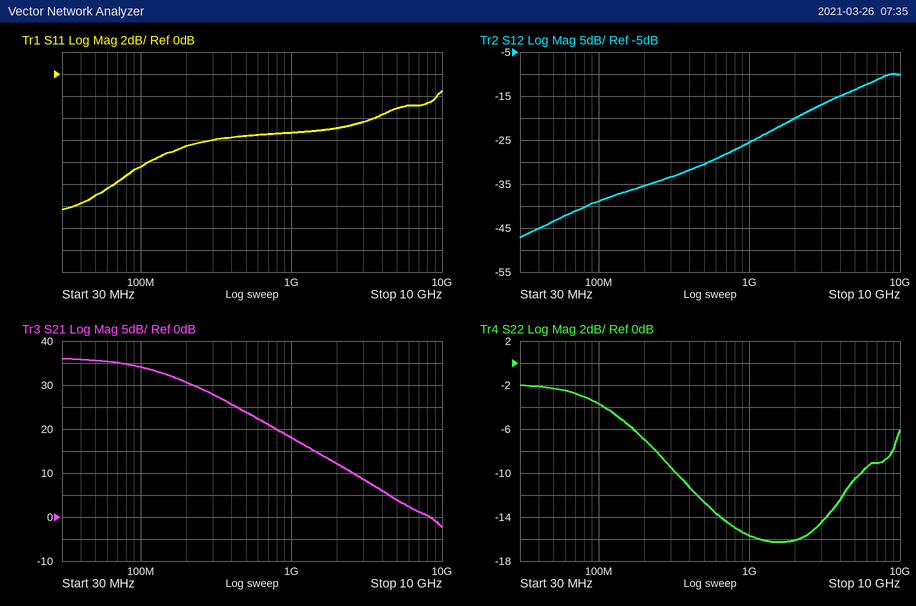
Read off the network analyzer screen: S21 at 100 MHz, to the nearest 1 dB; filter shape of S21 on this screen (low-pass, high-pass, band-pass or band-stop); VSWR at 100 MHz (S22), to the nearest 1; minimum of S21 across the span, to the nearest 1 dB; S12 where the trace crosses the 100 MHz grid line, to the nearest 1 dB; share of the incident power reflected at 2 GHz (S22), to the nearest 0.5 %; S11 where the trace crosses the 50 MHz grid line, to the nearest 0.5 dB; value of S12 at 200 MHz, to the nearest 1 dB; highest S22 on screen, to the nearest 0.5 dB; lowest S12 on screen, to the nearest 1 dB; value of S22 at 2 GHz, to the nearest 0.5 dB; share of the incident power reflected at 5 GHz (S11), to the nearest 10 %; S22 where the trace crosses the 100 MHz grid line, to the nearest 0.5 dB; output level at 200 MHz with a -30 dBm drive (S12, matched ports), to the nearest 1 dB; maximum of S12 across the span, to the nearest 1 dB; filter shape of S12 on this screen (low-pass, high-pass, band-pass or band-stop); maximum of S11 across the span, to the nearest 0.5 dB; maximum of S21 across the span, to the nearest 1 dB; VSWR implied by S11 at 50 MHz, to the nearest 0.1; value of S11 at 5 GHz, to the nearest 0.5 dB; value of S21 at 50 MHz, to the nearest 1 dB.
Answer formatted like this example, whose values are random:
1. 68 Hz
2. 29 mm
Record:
1. 34 dB
2. low-pass
3. 5
4. -2 dB
5. -39 dB
6. 2.5 %
7. -11.0 dB
8. -35 dB
9. -2.0 dB
10. -47 dB
11. -16.0 dB
12. 50 %
13. -3.5 dB
14. -65 dBm
15. -10 dB
16. high-pass
17. -1.5 dB
18. 36 dB
19. 1.8
20. -3.0 dB
21. 36 dB
